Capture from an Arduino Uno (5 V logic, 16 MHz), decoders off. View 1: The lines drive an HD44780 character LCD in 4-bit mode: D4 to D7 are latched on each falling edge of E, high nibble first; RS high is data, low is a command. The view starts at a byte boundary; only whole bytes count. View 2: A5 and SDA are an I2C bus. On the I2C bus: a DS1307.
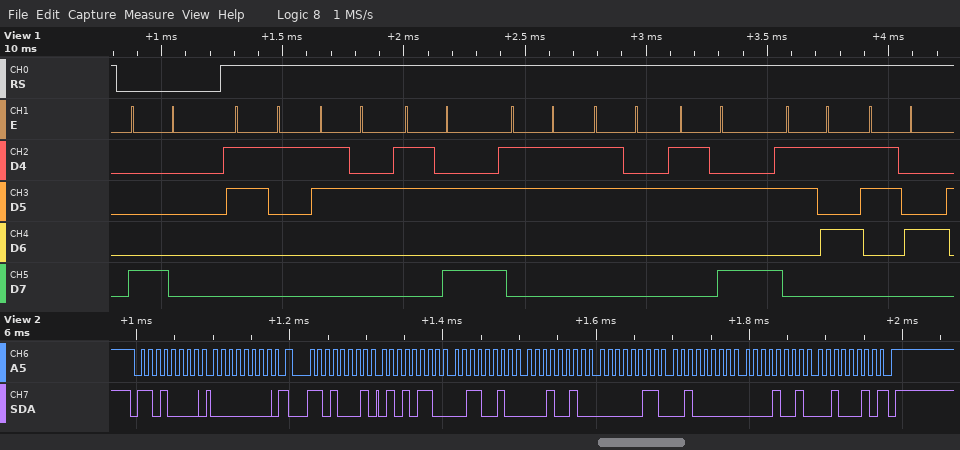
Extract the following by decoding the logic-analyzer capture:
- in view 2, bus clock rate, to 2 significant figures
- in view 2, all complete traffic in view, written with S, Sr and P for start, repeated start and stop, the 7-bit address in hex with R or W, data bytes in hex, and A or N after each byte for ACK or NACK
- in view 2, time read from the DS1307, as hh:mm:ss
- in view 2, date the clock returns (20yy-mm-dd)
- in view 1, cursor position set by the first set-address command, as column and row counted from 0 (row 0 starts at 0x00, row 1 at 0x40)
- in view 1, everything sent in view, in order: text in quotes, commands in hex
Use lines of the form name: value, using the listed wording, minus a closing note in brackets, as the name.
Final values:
in view 2, bus clock rate, to 2 significant figures: 100 kHz
in view 2, all complete traffic in view, written with S, Sr and P for start, repeated start and stop, the 7-bit address in hex with R or W, data bytes in hex, and A or N after each byte for ACK or NACK: S 68W A 00 A Sr 68R A 56 A 32 A 12 A 03 A 20 A 09 A 22 N P
in view 2, time read from the DS1307, as hh:mm:ss: 12:32:56
in view 2, date the clock returns: 2022-09-20
in view 1, cursor position set by the first set-address command, as column and row counted from 0: column 0, row 0
in view 1, everything sent in view, in order: text in quotes, commands in hex: 0x80 "12:32:54"
